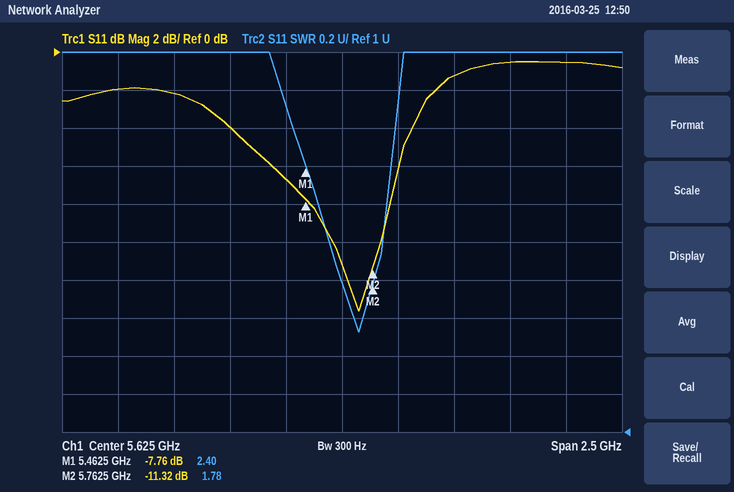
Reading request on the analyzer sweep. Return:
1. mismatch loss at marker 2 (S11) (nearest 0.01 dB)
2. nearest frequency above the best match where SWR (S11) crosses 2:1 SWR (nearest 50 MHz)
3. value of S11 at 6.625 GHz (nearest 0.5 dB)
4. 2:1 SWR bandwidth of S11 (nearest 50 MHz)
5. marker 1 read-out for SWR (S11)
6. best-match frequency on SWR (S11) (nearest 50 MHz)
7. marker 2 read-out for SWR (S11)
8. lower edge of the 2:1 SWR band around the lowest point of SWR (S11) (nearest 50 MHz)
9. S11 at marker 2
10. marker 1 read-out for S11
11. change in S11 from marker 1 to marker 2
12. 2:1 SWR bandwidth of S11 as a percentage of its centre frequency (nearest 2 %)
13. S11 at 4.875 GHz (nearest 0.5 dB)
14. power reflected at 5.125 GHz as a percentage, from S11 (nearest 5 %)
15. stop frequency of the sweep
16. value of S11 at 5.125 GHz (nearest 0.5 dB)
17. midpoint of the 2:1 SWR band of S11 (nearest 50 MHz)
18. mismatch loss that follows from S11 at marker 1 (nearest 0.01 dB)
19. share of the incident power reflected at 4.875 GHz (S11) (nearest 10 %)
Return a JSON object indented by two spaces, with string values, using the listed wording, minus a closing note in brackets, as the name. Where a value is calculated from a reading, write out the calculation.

{
  "mismatch loss at marker 2 (S11)": "−10 log10(1 − 10^(-11.32/10)) ≈ 0.33 dB",
  "nearest frequency above the best match where SWR (S11) crosses 2:1 SWR": "5.80 GHz",
  "value of S11 at 6.625 GHz": "-0.5 dB",
  "2:1 SWR bandwidth of S11": "5.80 GHz − 5.55 GHz = 250 MHz",
  "marker 1 read-out for SWR": "2.40",
  "best-match frequency on SWR (S11)": "5.70 GHz",
  "marker 2 read-out for SWR": "1.78",
  "lower edge of the 2:1 SWR band around the lowest point of SWR (S11)": "5.55 GHz",
  "S11 at marker 2": "-11.32 dB",
  "marker 1 read-out for S11": "-7.76 dB",
  "change in S11 from marker 1 to marker 2": "-11.32 − (-7.76) = -3.56 dB",
  "2:1 SWR bandwidth of S11 as a percentage of its centre frequency": "250 MHz / 5.675 GHz ≈ 4 %",
  "S11 at 4.875 GHz": "-2.0 dB",
  "power reflected at 5.125 GHz as a percentage, from S11": "10^(-4/10) ≈ 40 %",
  "stop frequency of the sweep": "6.875 GHz",
  "value of S11 at 5.125 GHz": "-4.0 dB",
  "midpoint of the 2:1 SWR band of S11": "5.70 GHz",
  "mismatch loss that follows from S11 at marker 1": "−10 log10(1 − 10^(-7.76/10)) ≈ 0.80 dB",
  "share of the incident power reflected at 4.875 GHz (S11)": "10^(-2/10) ≈ 63.1 %, so 60 % to the nearest 10 %"
}
